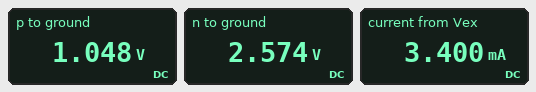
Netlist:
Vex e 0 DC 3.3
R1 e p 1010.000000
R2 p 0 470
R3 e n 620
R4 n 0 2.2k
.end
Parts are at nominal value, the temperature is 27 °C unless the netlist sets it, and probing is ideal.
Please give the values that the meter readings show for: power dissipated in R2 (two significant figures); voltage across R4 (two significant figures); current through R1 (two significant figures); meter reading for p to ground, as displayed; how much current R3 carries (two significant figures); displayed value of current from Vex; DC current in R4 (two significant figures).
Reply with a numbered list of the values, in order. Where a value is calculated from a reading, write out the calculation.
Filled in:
1. (1.048 V)^2 / 470 Ω = 2.3 mW
2. 2.574 V = 2.6 V
3. (3.3 V - 1.048 V) / 1.01 kΩ = 2.2 mA
4. 1.048 V
5. (3.3 V - 2.574 V) / 620 Ω = 1.2 mA
6. 3.400 mA
7. (2.574 V) / 2.2 kΩ = 1.2 mA
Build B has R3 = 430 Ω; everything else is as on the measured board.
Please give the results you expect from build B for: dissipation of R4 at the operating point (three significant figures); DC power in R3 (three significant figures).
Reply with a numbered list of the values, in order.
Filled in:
1. 3.46 mW
2. 677 µW
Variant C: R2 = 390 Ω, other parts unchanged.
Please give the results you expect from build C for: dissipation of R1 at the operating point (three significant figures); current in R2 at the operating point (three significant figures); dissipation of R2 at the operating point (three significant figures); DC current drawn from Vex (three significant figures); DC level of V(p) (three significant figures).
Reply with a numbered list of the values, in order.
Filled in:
1. 5.61 mW
2. 2.36 mA
3. 2.17 mW
4. 3.53 mA
5. 919 mV
